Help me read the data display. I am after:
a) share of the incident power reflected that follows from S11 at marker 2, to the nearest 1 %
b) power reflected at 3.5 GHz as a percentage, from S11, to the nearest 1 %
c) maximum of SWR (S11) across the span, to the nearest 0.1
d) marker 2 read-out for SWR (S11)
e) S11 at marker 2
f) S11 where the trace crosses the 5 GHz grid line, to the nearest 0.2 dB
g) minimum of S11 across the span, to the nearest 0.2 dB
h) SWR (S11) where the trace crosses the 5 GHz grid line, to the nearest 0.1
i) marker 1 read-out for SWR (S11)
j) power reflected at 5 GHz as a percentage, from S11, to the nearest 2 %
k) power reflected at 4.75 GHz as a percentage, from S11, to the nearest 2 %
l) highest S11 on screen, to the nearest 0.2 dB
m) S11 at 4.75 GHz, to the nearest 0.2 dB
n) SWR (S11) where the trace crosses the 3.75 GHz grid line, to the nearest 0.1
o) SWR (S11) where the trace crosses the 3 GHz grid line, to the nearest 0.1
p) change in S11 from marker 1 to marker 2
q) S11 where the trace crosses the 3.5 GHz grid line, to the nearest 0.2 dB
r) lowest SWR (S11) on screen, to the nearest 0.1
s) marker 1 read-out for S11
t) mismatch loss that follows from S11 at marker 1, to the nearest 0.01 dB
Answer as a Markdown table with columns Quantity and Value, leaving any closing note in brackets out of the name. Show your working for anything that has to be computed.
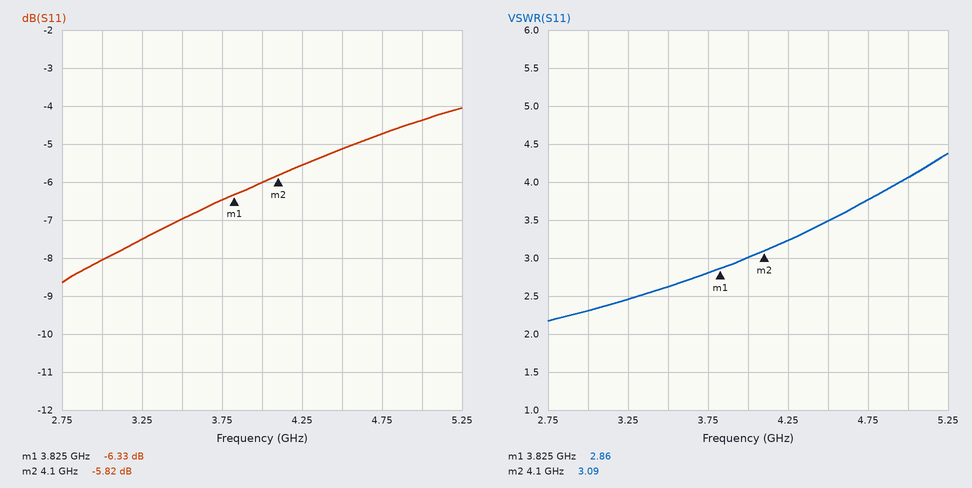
| Quantity | Value |
|---|---|
| share of the incident power reflected that follows from S11 at marker 2, to the nearest 1 % | 10^(-5.82/10) ≈ 26 % |
| power reflected at 3.5 GHz as a percentage, from S11, to the nearest 1 % | 10^(-7/10) ≈ 20 % |
| maximum of SWR (S11) across the span, to the nearest 0.1 | 4.4 |
| marker 2 read-out for SWR | 3.09 |
| S11 at marker 2 | -5.82 dB |
| S11 where the trace crosses the 5 GHz grid line, to the nearest 0.2 dB | -4.4 dB |
| minimum of S11 across the span, to the nearest 0.2 dB | -8.6 dB |
| SWR (S11) where the trace crosses the 5 GHz grid line, to the nearest 0.1 | 4.1 |
| marker 1 read-out for SWR | 2.86 |
| power reflected at 5 GHz as a percentage, from S11, to the nearest 2 % | 10^(-4.4/10) ≈ 36 % |
| power reflected at 4.75 GHz as a percentage, from S11, to the nearest 2 % | 10^(-4.8/10) ≈ 33.1 %, so 34 % to the nearest 2 % |
| highest S11 on screen, to the nearest 0.2 dB | -4.0 dB |
| S11 at 4.75 GHz, to the nearest 0.2 dB | -4.8 dB |
| SWR (S11) where the trace crosses the 3.75 GHz grid line, to the nearest 0.1 | 2.8 |
| SWR (S11) where the trace crosses the 3 GHz grid line, to the nearest 0.1 | 2.3 |
| change in S11 from marker 1 to marker 2 | -5.82 − (-6.33) = 0.51 dB |
| S11 where the trace crosses the 3.5 GHz grid line, to the nearest 0.2 dB | -7.0 dB |
| lowest SWR (S11) on screen, to the nearest 0.1 | 2.2 |
| marker 1 read-out for S11 | -6.33 dB |
| mismatch loss that follows from S11 at marker 1, to the nearest 0.01 dB | −10 log10(1 − 10^(-6.33/10)) ≈ 1.15 dB |
